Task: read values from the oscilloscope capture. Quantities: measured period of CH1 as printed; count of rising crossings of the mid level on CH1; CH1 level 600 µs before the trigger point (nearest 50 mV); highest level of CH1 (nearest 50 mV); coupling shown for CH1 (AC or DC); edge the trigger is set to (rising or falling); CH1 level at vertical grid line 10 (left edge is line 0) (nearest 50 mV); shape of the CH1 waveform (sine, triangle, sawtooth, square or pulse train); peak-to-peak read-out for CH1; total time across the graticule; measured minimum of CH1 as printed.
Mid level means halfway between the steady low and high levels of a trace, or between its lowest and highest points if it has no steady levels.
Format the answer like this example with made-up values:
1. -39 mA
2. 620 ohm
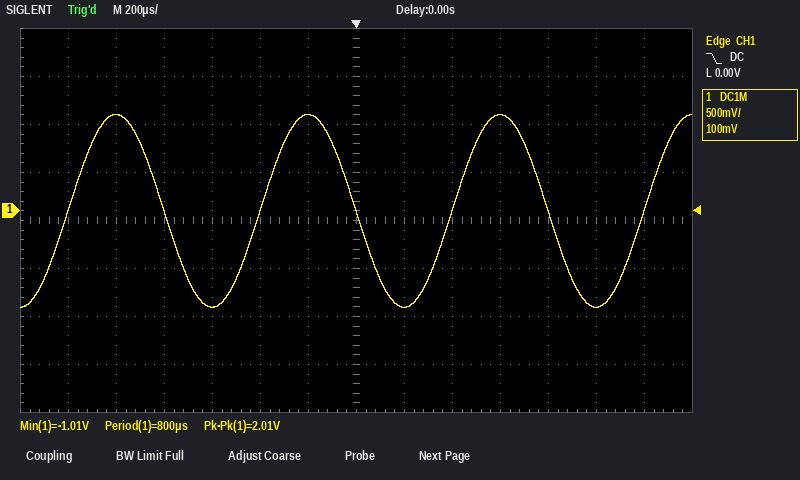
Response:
1. 800 µs
2. 4
3. -1.00 V
4. 1.00 V
5. DC
6. falling
7. 1.00 V
8. sine
9. 2.01 V
10. 2.8 ms
11. -1.01 V
